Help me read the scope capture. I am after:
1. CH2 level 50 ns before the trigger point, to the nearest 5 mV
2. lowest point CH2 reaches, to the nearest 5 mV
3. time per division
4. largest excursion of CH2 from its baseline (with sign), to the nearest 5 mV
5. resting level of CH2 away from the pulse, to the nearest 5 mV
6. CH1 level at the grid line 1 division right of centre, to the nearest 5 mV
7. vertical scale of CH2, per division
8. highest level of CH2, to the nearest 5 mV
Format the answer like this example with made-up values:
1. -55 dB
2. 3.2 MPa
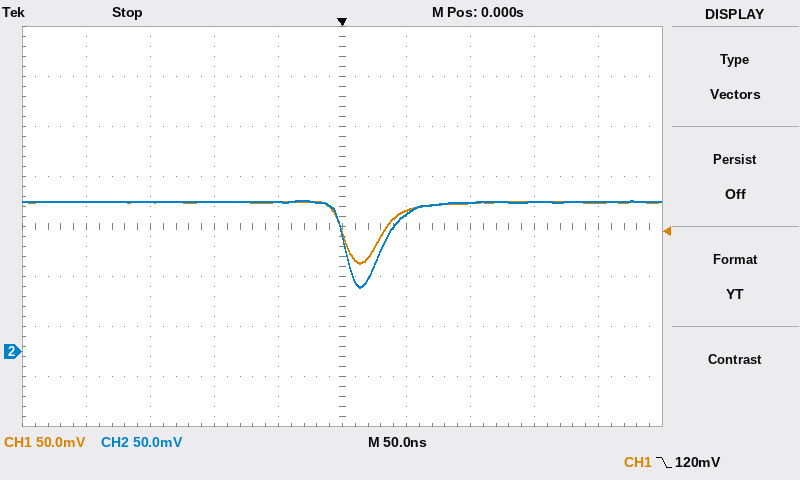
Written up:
1. 150 mV
2. 65 mV
3. 50 ns
4. -85 mV
5. 150 mV
6. 140 mV
7. 50 mV
8. 150 mV
